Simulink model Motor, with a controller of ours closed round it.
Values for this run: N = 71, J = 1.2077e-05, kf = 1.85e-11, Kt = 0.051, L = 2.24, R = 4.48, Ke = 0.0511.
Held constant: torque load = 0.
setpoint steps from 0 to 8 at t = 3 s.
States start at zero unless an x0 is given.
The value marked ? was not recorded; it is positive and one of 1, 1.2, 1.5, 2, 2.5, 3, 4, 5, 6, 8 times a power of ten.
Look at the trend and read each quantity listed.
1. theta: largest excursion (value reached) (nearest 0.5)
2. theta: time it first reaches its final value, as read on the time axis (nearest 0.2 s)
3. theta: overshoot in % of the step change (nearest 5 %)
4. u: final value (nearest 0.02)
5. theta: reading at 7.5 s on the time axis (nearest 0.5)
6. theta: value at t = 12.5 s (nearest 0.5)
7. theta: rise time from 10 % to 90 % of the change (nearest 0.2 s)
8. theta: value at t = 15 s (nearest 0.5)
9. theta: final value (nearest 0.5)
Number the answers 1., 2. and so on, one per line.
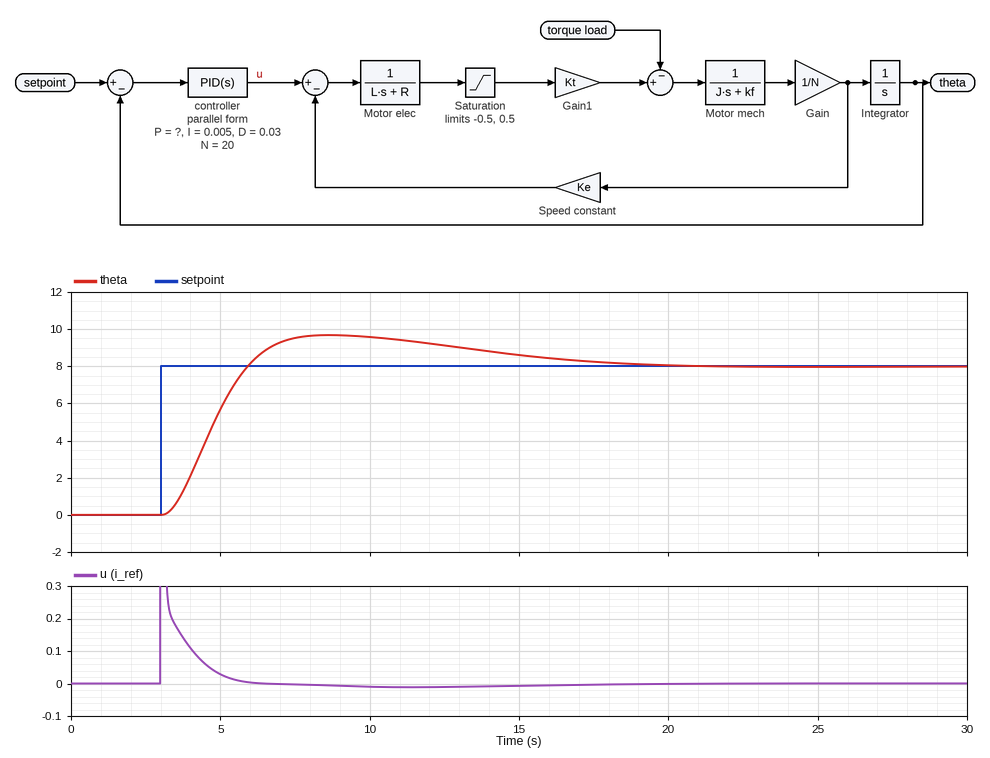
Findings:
1. 9.5
2. 6.0 s
3. 20 %
4. 0.00
5. 9.5
6. 9.0
7. 2.0 s
8. 8.5
9. 8.0
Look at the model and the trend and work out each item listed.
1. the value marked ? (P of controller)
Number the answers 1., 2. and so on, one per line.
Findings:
1. 0.03
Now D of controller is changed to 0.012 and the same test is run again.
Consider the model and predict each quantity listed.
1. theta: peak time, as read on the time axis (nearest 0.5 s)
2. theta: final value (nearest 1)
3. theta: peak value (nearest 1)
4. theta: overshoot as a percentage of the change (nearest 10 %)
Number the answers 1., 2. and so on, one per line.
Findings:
1. 8.5 s
2. 8
3. 11
4. 40 %
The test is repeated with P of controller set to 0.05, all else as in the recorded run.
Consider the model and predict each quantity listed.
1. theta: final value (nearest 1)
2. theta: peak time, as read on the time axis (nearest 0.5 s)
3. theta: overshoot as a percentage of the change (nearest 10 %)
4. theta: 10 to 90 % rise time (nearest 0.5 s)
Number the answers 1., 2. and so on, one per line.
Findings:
1. 8
2. 6.5 s
3. 30 %
4. 1.5 s
